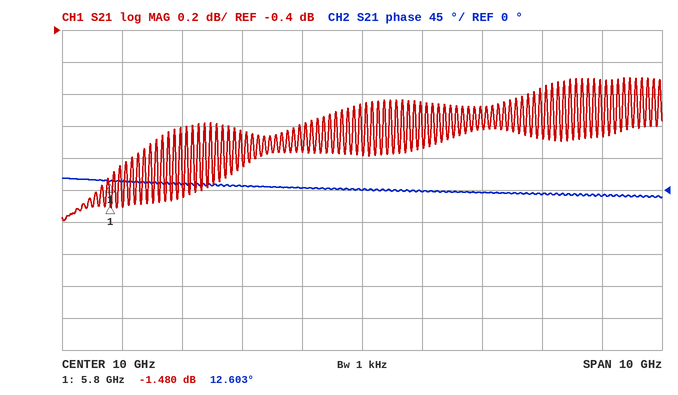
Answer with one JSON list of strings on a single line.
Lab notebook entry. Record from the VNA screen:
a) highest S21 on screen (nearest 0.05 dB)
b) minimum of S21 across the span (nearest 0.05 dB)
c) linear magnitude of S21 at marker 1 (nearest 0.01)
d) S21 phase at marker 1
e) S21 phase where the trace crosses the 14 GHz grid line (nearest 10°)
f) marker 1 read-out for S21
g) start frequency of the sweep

["-0.70 dB", "-1.60 dB", "0.84", "12.603°", "-10°", "-1.480 dB", "5 GHz"]
